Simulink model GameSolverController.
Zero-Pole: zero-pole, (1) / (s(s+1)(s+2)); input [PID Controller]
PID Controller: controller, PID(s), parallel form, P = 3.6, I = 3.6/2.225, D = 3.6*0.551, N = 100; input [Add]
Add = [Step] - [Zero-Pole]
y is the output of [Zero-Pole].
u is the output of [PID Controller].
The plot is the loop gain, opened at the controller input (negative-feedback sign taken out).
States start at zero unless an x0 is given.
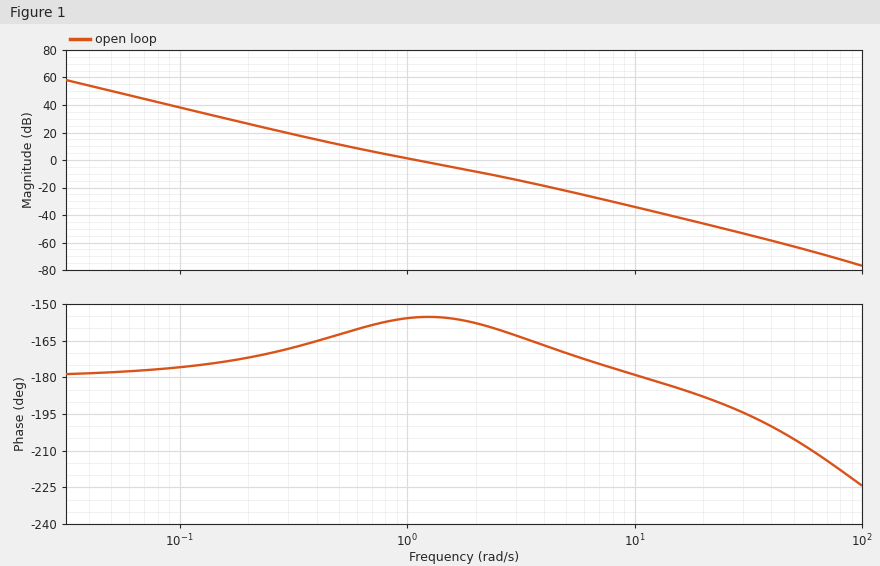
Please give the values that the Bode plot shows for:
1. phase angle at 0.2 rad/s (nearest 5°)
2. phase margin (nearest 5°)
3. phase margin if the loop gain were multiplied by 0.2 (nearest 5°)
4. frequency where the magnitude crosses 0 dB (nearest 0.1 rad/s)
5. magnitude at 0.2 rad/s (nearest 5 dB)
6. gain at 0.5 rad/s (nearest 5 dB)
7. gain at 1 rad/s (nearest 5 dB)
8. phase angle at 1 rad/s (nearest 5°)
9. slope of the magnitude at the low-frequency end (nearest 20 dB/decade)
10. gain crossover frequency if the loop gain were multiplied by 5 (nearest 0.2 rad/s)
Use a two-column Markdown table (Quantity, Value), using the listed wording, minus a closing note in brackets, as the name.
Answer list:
| Quantity | Value |
|---|---|
| phase angle at 0.2 rad/s | -170° |
| phase margin | 25° |
| phase margin if the loop gain were multiplied by 0.2 | 15° |
| frequency where the magnitude crosses 0 dB | 1.1 rad/s |
| magnitude at 0.2 rad/s | 25 dB |
| gain at 0.5 rad/s | 10 dB |
| gain at 1 rad/s | 0 dB |
| phase angle at 1 rad/s | -155° |
| slope of the magnitude at the low-frequency end | -40 dB/decade |
| gain crossover frequency if the loop gain were multiplied by 5 | 3.0 rad/s |
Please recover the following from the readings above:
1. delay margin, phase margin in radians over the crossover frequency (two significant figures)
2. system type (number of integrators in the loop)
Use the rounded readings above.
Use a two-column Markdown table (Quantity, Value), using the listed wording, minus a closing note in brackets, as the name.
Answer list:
| Quantity | Value |
|---|---|
| delay margin, phase margin in radians over the crossover frequency | 0.40 s |
| system type | 2 |
